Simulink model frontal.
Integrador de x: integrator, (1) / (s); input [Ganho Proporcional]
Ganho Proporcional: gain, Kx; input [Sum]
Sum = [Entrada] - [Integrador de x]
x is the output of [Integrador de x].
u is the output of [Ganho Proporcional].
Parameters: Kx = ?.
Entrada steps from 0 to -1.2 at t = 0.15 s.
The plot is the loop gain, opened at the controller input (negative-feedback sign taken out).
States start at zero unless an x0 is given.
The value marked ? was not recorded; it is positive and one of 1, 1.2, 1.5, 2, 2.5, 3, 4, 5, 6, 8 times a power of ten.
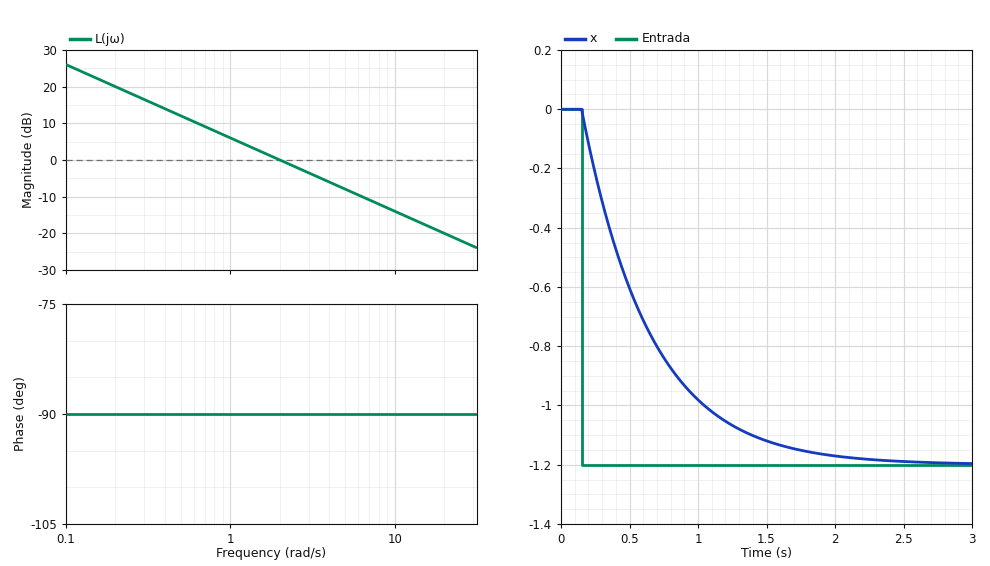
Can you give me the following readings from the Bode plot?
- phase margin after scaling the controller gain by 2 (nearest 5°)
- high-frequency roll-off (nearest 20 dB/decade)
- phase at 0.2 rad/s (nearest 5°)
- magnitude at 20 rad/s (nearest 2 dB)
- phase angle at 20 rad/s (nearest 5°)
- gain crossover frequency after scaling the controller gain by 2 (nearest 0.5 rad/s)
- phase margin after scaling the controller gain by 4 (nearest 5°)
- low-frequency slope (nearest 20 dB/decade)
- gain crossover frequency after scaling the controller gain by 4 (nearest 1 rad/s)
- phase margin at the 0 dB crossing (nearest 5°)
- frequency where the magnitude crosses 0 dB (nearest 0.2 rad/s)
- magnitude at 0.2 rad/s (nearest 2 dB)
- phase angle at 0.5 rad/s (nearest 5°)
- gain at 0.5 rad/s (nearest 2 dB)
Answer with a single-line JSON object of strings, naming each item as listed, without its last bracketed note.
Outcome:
{"phase margin after scaling the controller gain by 2": "90°", "high-frequency roll-off": "-20 dB/decade", "phase at 0.2 rad/s": "-90°", "magnitude at 20 rad/s": "-20 dB", "phase angle at 20 rad/s": "-90°", "gain crossover frequency after scaling the controller gain by 2": "4.0 rad/s", "phase margin after scaling the controller gain by 4": "90°", "low-frequency slope": "-20 dB/decade", "gain crossover frequency after scaling the controller gain by 4": "8 rad/s", "phase margin at the 0 dB crossing": "90°", "frequency where the magnitude crosses 0 dB": "2.0 rad/s", "magnitude at 0.2 rad/s": "20 dB", "phase angle at 0.5 rad/s": "-90°", "gain at 0.5 rad/s": "12 dB"}
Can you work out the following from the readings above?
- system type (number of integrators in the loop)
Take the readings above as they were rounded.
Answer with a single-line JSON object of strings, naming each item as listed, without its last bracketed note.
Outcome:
{"system type": "1"}
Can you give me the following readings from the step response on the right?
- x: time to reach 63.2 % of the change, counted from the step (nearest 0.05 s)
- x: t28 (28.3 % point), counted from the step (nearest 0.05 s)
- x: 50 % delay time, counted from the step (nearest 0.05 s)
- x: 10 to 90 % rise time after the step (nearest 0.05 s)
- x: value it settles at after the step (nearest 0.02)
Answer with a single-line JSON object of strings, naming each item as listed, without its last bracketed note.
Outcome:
{"x: time to reach 63.2 % of the change, counted from the step": "0.50 s", "x: t28 (28.3 % point), counted from the step": "0.15 s", "x: 50 % delay time, counted from the step": "0.35 s", "x: 10 to 90 % rise time after the step": "1.10 s", "x: value it settles at after the step": "-1.20"}
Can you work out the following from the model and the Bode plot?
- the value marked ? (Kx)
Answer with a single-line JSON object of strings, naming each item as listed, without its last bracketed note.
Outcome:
{"the value marked ?": "2"}
